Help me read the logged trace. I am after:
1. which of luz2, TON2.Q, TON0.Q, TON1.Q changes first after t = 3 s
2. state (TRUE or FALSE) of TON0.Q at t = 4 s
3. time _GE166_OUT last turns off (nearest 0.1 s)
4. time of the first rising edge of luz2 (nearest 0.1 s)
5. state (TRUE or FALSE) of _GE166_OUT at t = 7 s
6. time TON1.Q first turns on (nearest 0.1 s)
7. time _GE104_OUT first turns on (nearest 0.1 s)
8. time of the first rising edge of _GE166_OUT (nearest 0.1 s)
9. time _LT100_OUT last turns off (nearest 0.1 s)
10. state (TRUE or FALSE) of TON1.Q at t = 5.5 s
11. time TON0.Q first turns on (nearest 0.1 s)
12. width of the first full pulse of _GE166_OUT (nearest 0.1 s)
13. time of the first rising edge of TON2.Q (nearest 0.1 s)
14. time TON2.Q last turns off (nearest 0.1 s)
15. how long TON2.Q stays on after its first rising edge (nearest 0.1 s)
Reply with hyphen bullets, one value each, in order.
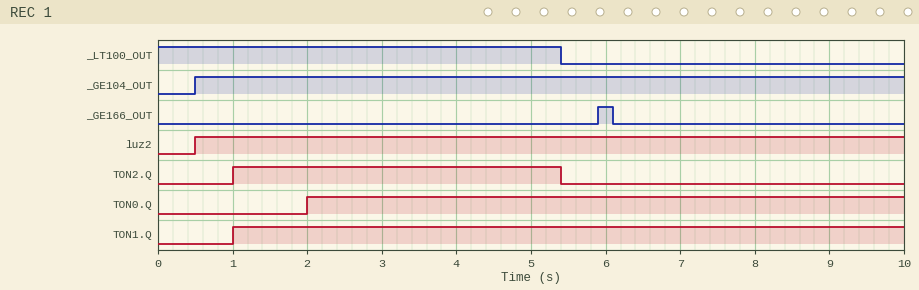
- TON2.Q
- TRUE
- 6.1 s
- 0.5 s
- FALSE
- 1.0 s
- 0.5 s
- 5.9 s
- 5.4 s
- TRUE
- 2.0 s
- 0.2 s
- 1.0 s
- 5.4 s
- 4.4 s
